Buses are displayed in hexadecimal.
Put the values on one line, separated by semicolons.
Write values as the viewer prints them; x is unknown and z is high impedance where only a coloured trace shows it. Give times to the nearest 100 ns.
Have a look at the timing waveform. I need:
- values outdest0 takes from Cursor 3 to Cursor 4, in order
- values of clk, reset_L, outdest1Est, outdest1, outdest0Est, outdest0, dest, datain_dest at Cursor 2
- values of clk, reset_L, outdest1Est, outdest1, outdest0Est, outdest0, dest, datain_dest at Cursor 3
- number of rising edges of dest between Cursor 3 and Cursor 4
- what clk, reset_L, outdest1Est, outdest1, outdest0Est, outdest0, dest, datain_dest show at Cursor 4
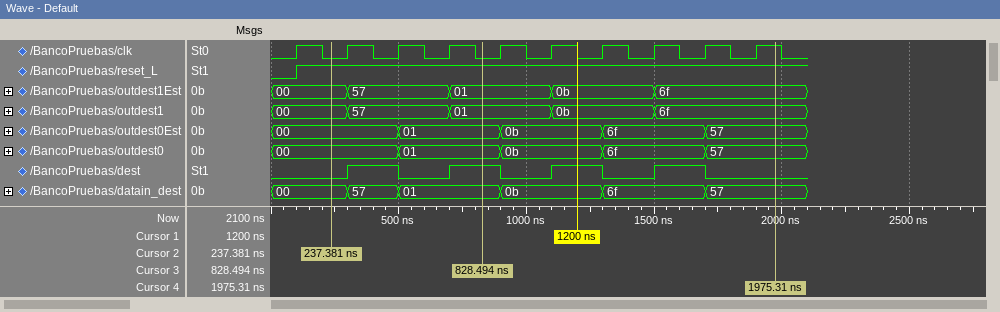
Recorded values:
01, 0b, 6f, 57; clk=0, reset_L=1, outdest1Est=00, outdest1=00, outdest0Est=00, outdest0=00, dest=0, datain_dest=00; clk=0, reset_L=1, outdest1Est=01, outdest1=01, outdest0Est=01, outdest0=01, dest=1, datain_dest=01; 2; clk=1, reset_L=1, outdest1Est=6f, outdest1=6f, outdest0Est=57, outdest0=57, dest=0, datain_dest=57
